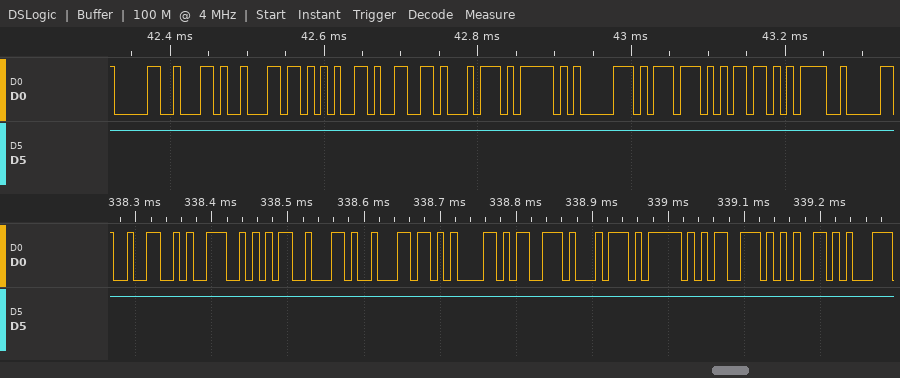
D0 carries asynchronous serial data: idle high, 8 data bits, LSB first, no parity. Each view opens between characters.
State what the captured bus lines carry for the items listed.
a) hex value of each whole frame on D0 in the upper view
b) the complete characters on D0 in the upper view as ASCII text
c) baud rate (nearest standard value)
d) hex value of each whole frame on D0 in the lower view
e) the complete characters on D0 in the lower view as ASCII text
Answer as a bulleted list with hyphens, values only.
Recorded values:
- 30, 2C, 6C, 65, 66, 74, 5F, 70, 77, 6D, 3D
- "0,left_pwm="
- 115200 baud
- 32, 39, 35, 2C, 6C, 61, 73, 74, 5F, 73, 65
- "295,last_se"
